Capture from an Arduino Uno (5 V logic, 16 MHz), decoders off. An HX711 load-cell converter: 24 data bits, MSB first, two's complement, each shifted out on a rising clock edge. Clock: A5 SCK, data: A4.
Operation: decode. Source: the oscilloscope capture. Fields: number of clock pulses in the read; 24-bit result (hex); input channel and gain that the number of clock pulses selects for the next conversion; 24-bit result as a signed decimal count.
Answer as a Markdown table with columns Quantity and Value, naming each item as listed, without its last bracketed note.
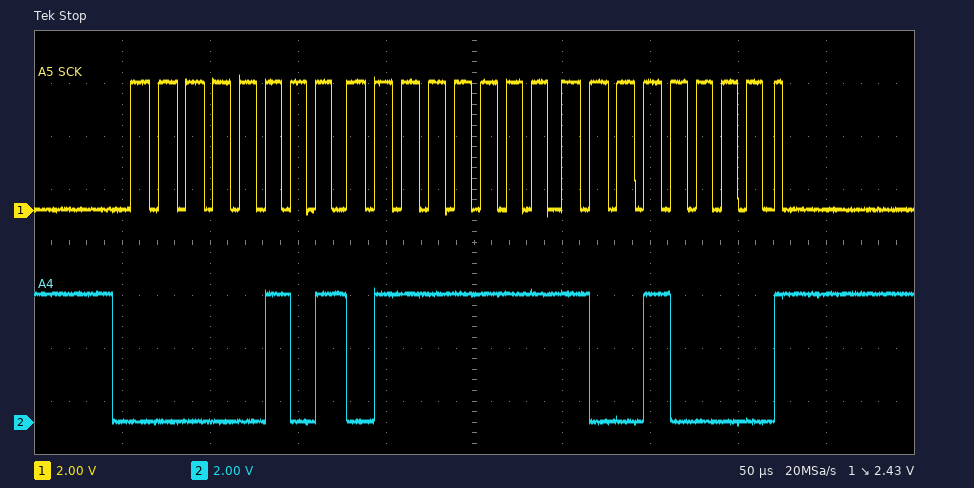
| Quantity | Value |
|---|---|
| number of clock pulses in the read | 25 |
| 24-bit result | 0x057F90 |
| input channel and gain that the number of clock pulses selects for the next conversion | channel A, gain 128 |
| 24-bit result as a signed decimal count | 360336 |
